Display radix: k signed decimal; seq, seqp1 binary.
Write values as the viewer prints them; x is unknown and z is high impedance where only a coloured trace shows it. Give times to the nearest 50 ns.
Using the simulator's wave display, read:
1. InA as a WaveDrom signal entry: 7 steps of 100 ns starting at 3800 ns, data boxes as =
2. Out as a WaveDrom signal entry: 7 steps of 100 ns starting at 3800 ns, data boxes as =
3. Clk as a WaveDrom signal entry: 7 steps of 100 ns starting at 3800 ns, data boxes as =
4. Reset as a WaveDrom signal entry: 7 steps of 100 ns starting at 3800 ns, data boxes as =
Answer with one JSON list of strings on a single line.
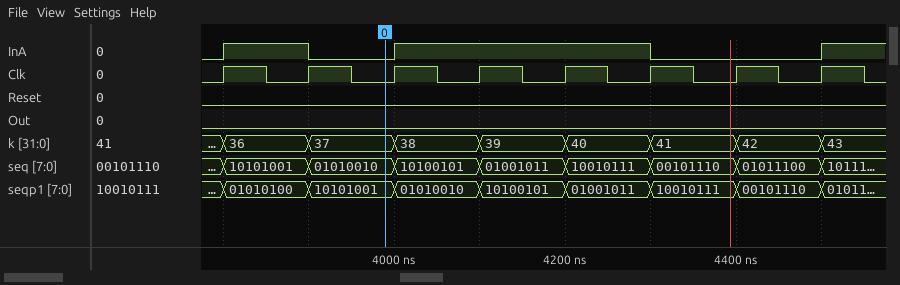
["{name: 'InA', wave: '101..0.'}", "{name: 'Out', wave: '0......'}", "{name: 'Clk', wave: 'p......'}", "{name: 'Reset', wave: '0......'}"]
